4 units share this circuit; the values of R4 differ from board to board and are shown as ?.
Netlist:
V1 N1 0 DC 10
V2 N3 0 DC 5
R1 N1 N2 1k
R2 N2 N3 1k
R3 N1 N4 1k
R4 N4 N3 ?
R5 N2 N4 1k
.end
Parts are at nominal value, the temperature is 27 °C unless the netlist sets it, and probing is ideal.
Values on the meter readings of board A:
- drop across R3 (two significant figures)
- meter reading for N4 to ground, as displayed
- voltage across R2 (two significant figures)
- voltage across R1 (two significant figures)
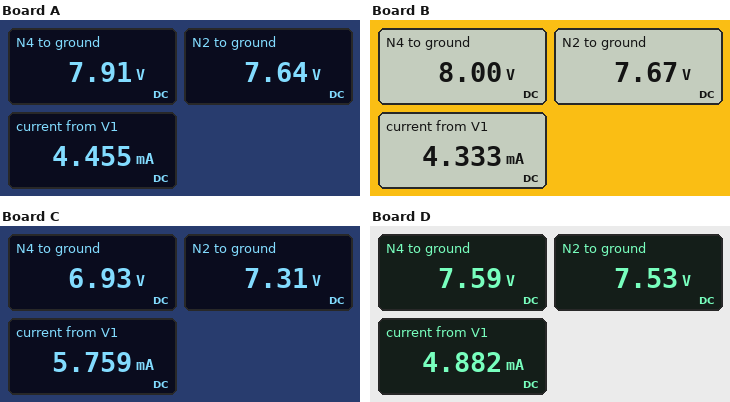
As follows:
2.1 V
7.91 V
2.6 V
2.4 V
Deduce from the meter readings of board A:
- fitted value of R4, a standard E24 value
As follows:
1.6 kΩ
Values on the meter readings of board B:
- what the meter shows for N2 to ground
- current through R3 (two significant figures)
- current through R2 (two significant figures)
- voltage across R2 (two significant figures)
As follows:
7.67 V
2.0 mA
2.7 mA
2.7 V
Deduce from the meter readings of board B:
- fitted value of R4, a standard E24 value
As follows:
1.8 kΩ
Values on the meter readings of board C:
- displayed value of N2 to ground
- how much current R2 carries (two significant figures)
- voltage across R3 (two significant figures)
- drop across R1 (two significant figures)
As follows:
7.31 V
2.3 mA
3.1 V
2.7 V
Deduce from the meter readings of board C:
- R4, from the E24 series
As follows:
560 Ω
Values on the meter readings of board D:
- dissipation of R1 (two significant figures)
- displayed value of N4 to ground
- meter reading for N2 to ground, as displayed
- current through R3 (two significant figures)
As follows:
6.1 mW
7.59 V
7.53 V
2.4 mA
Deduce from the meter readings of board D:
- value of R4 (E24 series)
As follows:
1.1 kΩ
